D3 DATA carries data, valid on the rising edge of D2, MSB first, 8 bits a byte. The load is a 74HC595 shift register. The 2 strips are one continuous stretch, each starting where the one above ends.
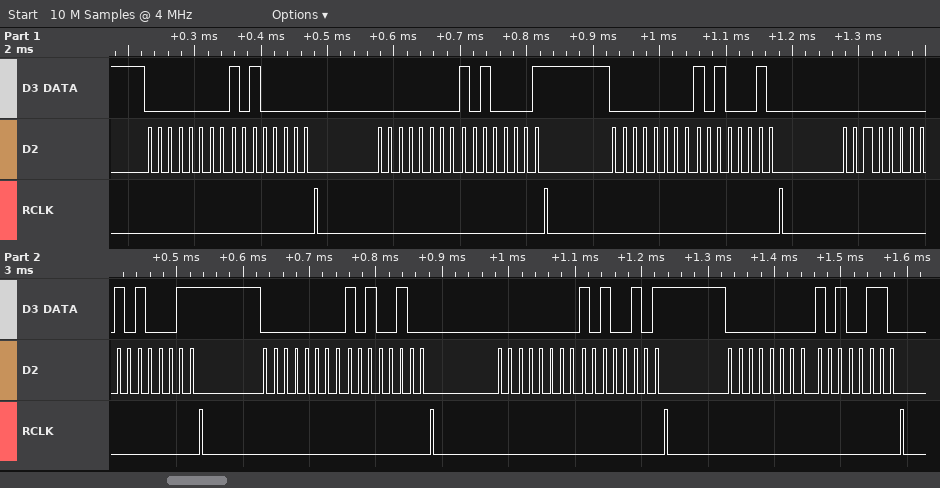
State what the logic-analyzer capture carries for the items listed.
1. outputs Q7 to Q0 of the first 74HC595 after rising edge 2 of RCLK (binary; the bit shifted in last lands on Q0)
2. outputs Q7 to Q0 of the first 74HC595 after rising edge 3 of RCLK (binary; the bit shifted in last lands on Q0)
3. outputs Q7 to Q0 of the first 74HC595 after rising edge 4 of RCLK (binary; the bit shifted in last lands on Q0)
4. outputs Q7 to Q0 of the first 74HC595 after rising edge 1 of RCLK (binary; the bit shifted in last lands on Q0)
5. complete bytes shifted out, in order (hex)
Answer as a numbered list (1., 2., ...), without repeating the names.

1. 10100001
2. 10100010
3. 10100011
4. 10100000
5. 0x00 0xA0 0x00 0xA1 0x00 0xA2 0x00 0xA3 0x00 0xA4 0x00 0xA5 0x00 0xA6
